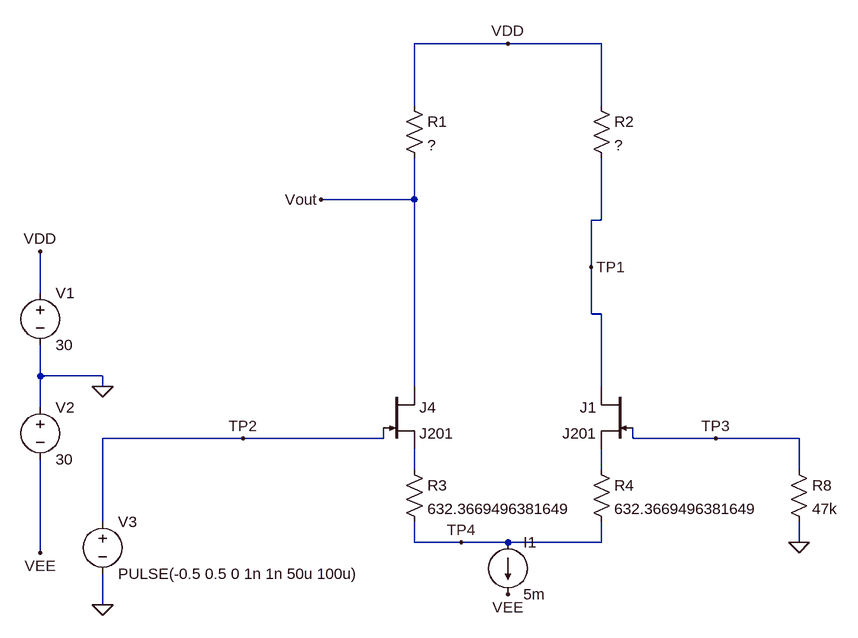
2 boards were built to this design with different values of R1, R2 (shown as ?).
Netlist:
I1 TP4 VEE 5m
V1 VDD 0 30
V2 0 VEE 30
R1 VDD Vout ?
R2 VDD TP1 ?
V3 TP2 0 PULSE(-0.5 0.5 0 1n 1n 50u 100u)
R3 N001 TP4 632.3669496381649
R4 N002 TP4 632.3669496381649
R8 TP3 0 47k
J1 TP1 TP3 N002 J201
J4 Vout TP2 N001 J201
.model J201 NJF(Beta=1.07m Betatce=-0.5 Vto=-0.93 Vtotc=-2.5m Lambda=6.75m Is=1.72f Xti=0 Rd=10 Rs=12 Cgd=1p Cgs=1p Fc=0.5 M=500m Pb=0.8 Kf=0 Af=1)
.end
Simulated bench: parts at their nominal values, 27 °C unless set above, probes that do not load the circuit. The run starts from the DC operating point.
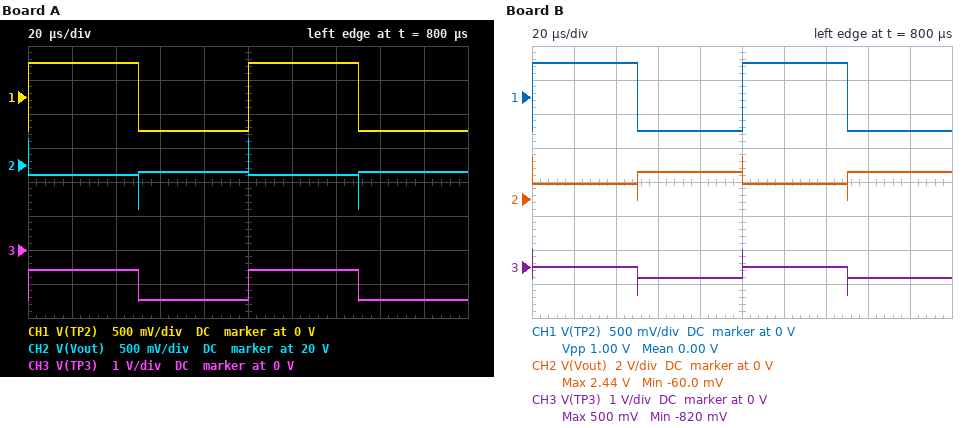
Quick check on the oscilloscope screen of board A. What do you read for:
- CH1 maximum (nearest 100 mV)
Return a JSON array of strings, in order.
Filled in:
["500 mV"]
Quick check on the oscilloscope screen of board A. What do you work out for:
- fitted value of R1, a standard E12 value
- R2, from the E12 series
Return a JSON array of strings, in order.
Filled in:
["3.3 kΩ", "18 kΩ"]
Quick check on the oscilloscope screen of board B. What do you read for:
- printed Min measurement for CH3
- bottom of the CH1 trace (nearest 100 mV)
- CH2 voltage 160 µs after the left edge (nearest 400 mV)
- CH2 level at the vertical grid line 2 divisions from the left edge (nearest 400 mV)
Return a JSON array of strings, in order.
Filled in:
["-820 mV", "-500 mV", "1.6 V", "800 mV"]
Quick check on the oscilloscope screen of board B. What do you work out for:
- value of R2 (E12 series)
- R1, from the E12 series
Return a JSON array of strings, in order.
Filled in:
["6.8 kΩ", "12 kΩ"]
